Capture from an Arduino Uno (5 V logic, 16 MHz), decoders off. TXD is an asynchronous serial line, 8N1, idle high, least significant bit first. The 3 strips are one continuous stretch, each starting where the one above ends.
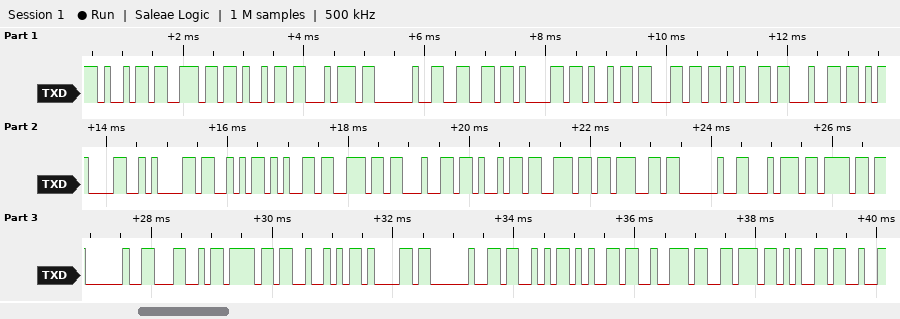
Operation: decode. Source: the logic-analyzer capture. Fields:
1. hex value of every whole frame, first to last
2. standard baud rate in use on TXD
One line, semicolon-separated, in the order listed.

69 6E 69 74 20 66 61 69 6C 65 64 0D 0A 53 65 6E 64 69 6E 67 20 74 6F 20 4C 6F 52 61 20 53 65 72 76 65; 9600 baud
